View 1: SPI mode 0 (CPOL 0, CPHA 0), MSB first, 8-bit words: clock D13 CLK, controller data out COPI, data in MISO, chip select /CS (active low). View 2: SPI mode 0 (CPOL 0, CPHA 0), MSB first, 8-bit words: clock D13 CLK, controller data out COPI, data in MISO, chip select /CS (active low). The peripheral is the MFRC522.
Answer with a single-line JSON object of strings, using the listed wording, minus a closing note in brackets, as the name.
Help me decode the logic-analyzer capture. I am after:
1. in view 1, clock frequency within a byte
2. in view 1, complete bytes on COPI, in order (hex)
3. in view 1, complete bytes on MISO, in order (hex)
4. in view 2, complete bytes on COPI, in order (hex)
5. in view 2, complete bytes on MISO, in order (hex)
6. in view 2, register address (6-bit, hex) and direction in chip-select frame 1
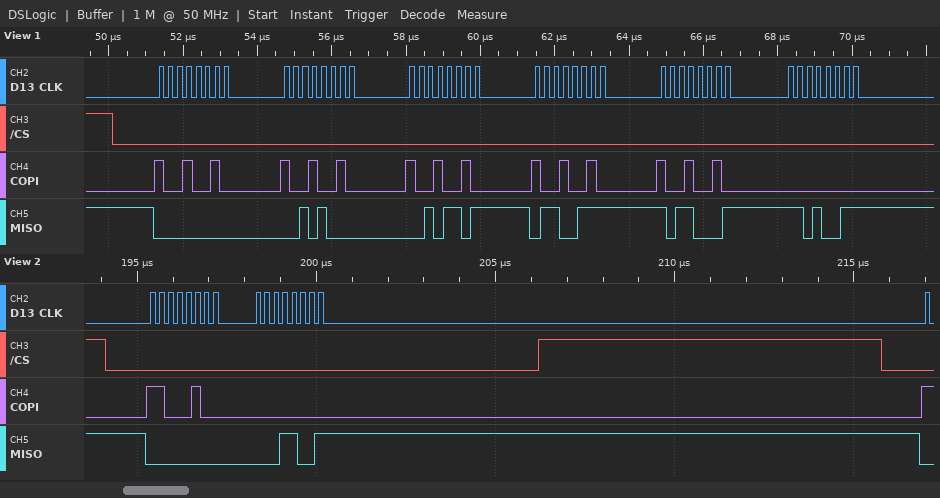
{"in view 1, clock frequency within a byte": "4 MHz", "in view 1, complete bytes on COPI, in order": "92 92 92 92 92 00", "in view 1, complete bytes on MISO, in order": "00 28 2D 67 B1 D3", "in view 2, complete bytes on COPI, in order": "C4 00", "in view 2, complete bytes on MISO, in order": "00 19", "in view 2, register address (6-bit, hex) and direction in chip-select frame 1": "0x22 read"}
